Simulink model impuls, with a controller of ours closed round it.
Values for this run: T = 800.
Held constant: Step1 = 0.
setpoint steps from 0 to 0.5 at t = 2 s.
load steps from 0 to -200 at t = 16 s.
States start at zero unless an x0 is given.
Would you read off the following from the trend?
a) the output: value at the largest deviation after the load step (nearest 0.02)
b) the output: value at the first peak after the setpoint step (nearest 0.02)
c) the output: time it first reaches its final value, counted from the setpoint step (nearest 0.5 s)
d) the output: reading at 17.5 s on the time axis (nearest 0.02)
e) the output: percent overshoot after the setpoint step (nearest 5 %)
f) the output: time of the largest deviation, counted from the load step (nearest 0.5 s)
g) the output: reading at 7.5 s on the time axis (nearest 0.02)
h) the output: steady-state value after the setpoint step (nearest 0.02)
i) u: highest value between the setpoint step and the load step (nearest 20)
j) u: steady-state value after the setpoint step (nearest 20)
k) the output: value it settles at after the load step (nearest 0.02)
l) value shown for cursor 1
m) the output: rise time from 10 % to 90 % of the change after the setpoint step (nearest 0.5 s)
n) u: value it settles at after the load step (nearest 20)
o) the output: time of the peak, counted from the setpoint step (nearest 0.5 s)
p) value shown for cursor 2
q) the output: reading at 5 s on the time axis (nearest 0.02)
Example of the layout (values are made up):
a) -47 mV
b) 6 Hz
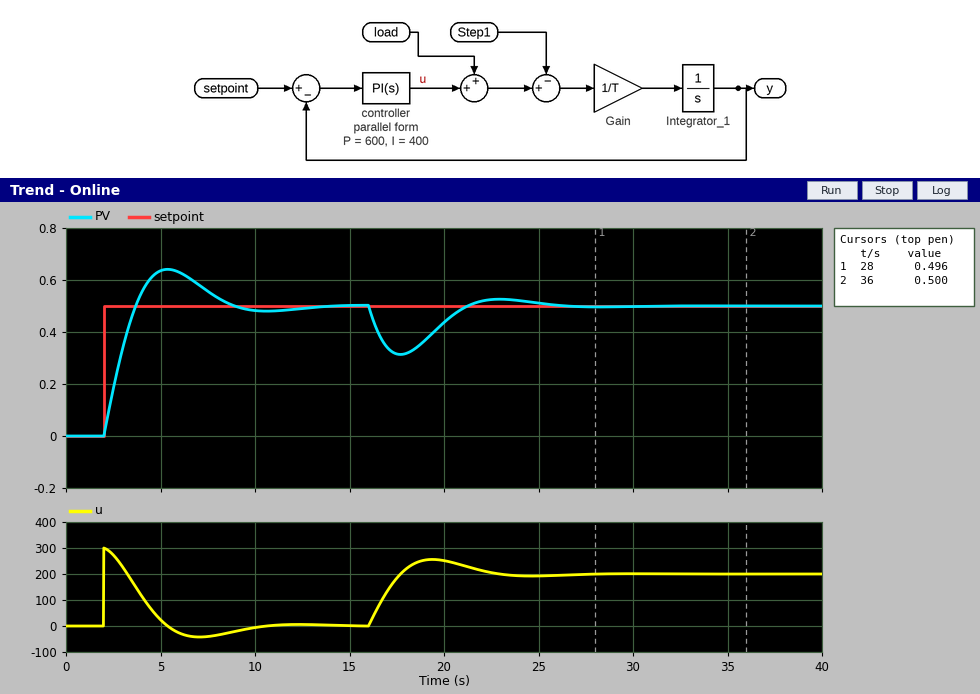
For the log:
a) 0.32
b) 0.64
c) 1.5 s
d) 0.32
e) 30 %
f) 1.5 s
g) 0.56
h) 0.50
i) 300
j) 0
k) 0.50
l) 0.496
m) 1.5 s
n) 200
o) 3.5 s
p) 0.500
q) 0.64
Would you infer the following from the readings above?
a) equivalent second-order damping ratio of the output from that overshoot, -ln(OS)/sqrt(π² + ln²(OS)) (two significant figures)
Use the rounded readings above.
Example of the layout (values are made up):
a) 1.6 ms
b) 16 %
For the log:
a) 0.36
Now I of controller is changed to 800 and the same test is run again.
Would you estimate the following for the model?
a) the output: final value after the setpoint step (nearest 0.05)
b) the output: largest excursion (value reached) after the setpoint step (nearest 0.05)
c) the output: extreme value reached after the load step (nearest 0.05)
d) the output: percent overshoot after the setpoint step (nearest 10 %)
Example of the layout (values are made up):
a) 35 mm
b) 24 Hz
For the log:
a) 0.50
b) 0.70
c) 0.35
d) 40 %
